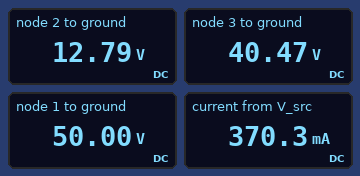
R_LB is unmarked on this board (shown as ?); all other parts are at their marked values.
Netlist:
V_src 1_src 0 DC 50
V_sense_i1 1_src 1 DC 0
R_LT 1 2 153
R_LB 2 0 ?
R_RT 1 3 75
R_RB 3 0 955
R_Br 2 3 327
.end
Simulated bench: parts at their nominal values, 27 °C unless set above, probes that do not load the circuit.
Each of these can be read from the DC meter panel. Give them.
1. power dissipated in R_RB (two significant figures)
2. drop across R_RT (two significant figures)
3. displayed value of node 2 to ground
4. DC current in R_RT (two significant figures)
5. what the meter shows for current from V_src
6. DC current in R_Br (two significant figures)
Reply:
1.7 W
9.5 V
12.79 V
130 mA
370.3 mA
85 mA
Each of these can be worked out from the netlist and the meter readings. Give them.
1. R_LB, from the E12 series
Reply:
39 Ω
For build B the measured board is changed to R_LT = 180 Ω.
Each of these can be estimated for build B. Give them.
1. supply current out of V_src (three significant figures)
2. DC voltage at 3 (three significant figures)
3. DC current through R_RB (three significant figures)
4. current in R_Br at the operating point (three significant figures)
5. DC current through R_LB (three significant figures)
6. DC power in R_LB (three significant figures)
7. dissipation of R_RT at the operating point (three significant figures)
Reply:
342 mA
40.3 V
42.2 mA
87.4 mA
300 mA
3.51 W
1.26 W
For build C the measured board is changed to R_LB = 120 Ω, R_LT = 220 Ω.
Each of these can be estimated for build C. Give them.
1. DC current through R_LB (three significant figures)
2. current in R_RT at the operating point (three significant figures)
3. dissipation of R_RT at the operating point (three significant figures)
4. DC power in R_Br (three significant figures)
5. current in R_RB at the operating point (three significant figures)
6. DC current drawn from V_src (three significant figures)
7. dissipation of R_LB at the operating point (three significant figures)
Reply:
186 mA
105 mA
822 mW
1.20 W
44.1 mA
230 mA
4.16 W
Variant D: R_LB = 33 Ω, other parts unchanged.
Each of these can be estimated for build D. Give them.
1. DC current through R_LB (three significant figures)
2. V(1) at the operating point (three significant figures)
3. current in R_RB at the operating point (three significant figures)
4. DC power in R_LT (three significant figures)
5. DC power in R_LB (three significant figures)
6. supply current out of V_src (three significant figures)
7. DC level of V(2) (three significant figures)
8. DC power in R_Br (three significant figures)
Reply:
342 mA
50.0 V
42.1 mA
9.80 W
3.85 W
384 mA
11.3 V
2.56 W
